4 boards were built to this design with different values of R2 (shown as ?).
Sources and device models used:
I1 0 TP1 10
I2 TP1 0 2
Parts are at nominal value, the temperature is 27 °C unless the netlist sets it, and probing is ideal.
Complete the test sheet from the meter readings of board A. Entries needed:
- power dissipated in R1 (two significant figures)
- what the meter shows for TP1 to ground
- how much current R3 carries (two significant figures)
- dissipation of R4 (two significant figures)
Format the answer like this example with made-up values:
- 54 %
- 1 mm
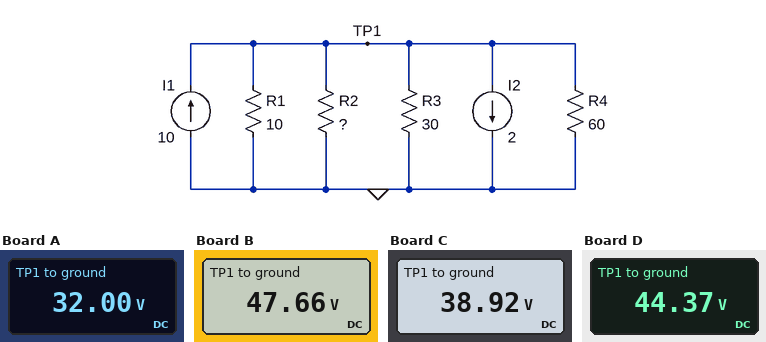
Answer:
- 100 W
- 32.00 V
- 1.1 A
- 17 W
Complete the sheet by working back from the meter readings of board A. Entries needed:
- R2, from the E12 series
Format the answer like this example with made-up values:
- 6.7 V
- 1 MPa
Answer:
- 10 Ω
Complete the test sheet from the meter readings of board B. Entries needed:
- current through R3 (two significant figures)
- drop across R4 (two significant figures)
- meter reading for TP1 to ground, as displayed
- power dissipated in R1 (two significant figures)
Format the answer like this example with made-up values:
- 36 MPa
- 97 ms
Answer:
- 1.6 A
- 48 V
- 47.66 V
- 230 W
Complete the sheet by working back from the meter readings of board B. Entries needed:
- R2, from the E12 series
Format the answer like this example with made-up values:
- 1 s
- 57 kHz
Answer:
- 56 Ω
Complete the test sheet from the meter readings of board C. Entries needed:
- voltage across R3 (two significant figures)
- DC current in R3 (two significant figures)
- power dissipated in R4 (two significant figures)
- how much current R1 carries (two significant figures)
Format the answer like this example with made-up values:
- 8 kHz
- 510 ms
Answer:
- 39 V
- 1.3 A
- 25 W
- 3.9 A
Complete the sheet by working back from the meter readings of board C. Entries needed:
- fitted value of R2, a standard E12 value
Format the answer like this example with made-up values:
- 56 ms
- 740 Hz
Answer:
- 18 Ω
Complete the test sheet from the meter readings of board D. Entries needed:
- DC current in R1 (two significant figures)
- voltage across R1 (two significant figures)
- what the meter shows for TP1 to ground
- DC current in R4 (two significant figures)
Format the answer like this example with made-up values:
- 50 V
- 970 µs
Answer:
- 4.4 A
- 44 V
- 44.37 V
- 740 mA
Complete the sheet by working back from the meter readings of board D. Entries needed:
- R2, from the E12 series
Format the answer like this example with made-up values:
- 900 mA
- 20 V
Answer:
- 33 Ω
